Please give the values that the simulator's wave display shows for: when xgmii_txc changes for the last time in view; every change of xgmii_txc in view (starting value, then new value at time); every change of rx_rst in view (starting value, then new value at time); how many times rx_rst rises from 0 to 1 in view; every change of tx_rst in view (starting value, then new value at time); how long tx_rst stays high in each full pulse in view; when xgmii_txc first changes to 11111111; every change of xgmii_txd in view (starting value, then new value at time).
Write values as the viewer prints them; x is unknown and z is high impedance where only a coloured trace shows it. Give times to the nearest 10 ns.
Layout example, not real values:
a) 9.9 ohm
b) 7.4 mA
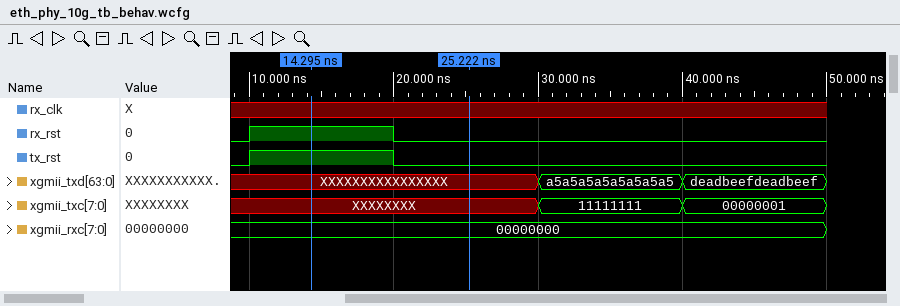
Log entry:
a) 40 ns
b) XXXXXXXX, 11111111 at 30 ns, 00000001 at 40 ns
c) 0, 1 at 10 ns, 0 at 20 ns
d) 1
e) 0, 1 at 10 ns, 0 at 20 ns
f) 10 ns
g) 30 ns
h) XXXXXXXXXXXXXXXX, a5a5a5a5a5a5a5a5 at 30 ns, deadbeefdeadbeef at 40 ns
